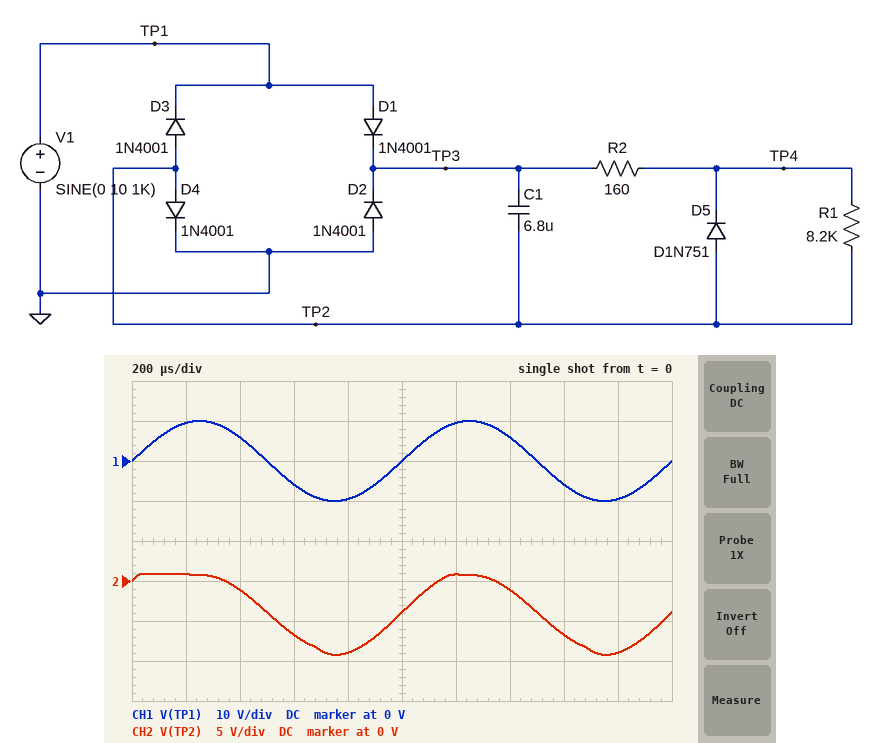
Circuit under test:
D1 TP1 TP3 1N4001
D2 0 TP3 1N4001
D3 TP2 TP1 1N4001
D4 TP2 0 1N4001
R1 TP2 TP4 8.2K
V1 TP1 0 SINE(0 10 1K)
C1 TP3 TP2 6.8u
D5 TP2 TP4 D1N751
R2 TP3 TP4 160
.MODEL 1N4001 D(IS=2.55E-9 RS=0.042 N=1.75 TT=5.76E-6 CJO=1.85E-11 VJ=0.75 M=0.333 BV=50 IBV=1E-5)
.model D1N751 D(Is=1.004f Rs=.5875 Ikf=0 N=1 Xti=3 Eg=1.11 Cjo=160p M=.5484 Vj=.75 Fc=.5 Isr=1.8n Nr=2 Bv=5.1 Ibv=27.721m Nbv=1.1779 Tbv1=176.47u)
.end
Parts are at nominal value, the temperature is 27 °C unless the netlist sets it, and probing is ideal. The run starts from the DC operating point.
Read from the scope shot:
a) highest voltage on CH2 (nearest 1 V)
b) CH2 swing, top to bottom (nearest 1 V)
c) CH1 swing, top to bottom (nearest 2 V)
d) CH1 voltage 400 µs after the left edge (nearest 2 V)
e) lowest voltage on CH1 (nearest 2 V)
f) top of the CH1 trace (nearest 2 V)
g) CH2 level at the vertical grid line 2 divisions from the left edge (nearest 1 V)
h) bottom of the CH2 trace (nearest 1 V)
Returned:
1 V
10 V
20 V
6 V
-10 V
10 V
-1 V
-9 V
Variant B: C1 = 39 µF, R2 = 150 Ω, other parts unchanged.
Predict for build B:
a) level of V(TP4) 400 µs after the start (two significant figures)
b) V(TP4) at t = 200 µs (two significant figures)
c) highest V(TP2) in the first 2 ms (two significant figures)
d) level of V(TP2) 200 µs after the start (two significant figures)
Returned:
3.9 V
6.0 V
1.0 V
930 mV
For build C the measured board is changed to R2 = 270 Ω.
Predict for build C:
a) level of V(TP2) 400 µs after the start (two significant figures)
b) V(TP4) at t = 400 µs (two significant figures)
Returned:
-1.2 V
3.9 V
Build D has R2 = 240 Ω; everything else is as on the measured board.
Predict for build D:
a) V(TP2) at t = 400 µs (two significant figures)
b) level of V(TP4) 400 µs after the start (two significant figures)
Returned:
-1.2 V
3.9 V
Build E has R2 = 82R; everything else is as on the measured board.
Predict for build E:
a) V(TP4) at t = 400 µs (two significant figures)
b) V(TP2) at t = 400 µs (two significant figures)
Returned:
4.2 V
-950 mV
